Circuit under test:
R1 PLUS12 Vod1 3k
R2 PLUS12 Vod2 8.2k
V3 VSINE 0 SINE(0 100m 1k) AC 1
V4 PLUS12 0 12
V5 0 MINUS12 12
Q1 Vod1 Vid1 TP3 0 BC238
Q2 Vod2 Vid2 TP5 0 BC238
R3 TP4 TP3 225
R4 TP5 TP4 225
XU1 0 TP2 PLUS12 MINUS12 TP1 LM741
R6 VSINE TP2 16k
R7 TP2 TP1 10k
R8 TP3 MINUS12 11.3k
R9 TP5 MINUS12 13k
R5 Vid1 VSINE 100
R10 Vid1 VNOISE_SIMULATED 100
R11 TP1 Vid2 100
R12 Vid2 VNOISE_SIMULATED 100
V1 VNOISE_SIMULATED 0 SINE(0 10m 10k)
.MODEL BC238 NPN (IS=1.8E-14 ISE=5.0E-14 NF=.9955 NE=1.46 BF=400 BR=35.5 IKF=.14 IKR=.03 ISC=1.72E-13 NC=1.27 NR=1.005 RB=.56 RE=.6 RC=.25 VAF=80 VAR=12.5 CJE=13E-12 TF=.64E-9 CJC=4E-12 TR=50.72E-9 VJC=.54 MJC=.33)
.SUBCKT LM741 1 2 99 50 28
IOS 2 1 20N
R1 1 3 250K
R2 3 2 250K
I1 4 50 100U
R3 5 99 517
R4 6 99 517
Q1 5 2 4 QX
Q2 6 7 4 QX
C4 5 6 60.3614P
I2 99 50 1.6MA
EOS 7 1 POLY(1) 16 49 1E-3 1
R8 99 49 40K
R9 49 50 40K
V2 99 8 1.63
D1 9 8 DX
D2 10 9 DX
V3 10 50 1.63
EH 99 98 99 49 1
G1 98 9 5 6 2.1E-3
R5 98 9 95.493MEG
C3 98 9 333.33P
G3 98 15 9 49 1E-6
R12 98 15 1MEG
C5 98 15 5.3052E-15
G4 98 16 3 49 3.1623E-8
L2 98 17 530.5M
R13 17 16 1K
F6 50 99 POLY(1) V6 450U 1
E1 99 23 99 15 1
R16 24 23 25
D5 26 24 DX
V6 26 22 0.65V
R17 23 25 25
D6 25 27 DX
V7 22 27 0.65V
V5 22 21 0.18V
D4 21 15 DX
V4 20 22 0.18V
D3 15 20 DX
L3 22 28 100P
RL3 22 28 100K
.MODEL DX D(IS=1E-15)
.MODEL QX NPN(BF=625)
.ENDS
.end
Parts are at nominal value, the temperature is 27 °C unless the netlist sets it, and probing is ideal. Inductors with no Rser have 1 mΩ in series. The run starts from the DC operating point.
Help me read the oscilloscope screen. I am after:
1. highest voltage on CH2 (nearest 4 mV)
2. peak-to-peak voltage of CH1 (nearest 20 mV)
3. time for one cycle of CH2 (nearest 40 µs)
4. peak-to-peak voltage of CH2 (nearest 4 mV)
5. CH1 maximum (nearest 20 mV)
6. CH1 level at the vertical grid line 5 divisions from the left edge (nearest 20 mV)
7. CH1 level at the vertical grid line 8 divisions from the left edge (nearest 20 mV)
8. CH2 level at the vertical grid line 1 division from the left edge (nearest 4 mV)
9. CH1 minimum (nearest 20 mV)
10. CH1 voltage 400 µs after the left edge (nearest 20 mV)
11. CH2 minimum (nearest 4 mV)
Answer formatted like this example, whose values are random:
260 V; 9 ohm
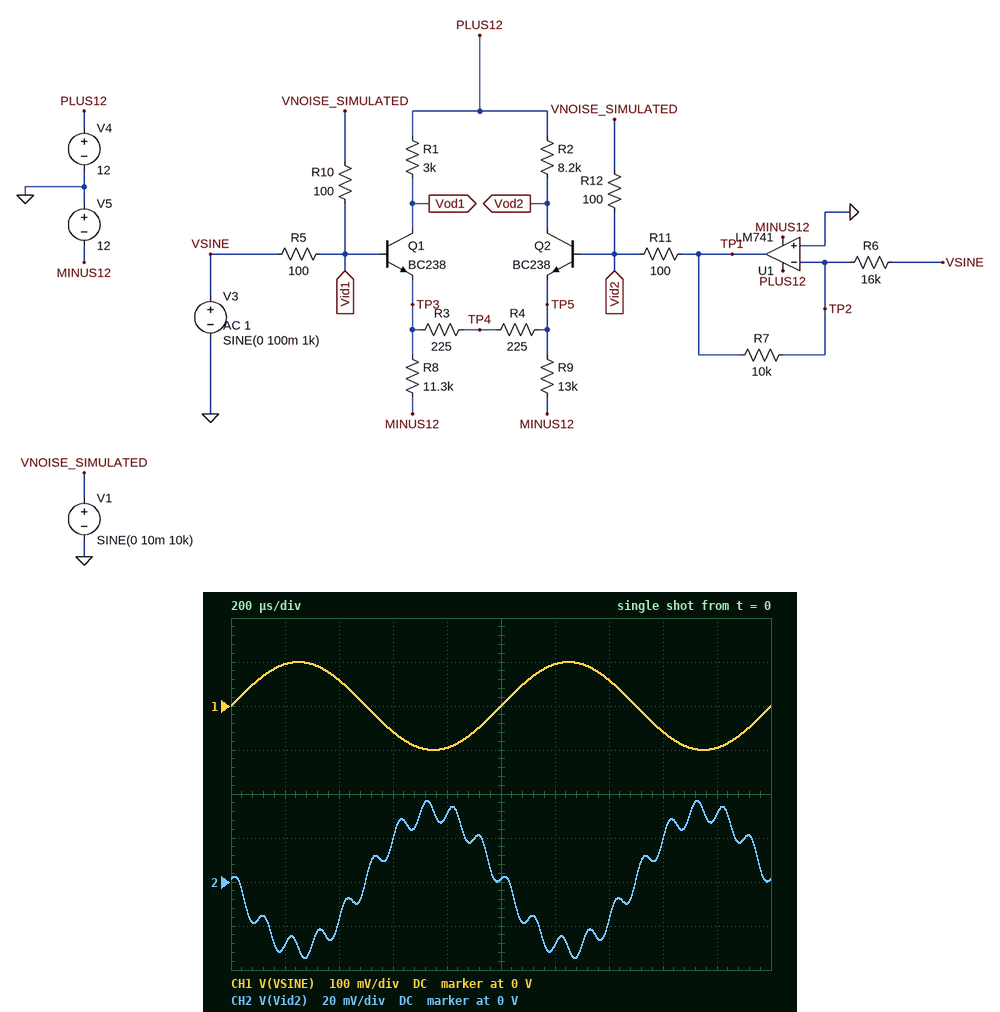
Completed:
36 mV; 200 mV; 1.00 ms; 72 mV; 100 mV; 0 V; -60 mV; -28 mV; -100 mV; 60 mV; -36 mV
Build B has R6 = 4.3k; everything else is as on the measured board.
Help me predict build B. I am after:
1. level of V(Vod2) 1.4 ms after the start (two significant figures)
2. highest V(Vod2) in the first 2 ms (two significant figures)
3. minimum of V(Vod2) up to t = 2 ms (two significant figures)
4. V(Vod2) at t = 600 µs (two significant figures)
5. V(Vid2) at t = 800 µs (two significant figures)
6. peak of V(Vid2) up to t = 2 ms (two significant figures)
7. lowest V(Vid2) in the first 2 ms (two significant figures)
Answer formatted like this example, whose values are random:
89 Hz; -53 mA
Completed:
6.4 V; 7.5 V; 2.1 V; 3.2 V; 110 mV; 120 mV; -120 mV
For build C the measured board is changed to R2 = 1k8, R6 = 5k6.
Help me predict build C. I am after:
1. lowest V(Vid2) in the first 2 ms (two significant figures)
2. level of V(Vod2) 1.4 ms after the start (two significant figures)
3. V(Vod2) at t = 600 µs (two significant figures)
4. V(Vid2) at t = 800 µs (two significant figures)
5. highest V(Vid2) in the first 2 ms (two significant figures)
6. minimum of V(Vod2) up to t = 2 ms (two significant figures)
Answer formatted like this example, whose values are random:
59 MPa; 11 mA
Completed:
-92 mV; 11 V; 10 V; 87 mV; 95 mV; 9.9 V
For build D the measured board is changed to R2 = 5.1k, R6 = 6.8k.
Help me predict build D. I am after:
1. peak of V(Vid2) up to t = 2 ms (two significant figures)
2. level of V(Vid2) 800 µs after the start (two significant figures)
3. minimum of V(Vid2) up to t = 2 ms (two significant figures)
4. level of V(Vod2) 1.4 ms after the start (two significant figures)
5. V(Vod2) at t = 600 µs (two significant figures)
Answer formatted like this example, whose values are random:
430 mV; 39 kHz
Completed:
79 mV; 72 mV; -76 mV; 8.2 V; 6.8 V
